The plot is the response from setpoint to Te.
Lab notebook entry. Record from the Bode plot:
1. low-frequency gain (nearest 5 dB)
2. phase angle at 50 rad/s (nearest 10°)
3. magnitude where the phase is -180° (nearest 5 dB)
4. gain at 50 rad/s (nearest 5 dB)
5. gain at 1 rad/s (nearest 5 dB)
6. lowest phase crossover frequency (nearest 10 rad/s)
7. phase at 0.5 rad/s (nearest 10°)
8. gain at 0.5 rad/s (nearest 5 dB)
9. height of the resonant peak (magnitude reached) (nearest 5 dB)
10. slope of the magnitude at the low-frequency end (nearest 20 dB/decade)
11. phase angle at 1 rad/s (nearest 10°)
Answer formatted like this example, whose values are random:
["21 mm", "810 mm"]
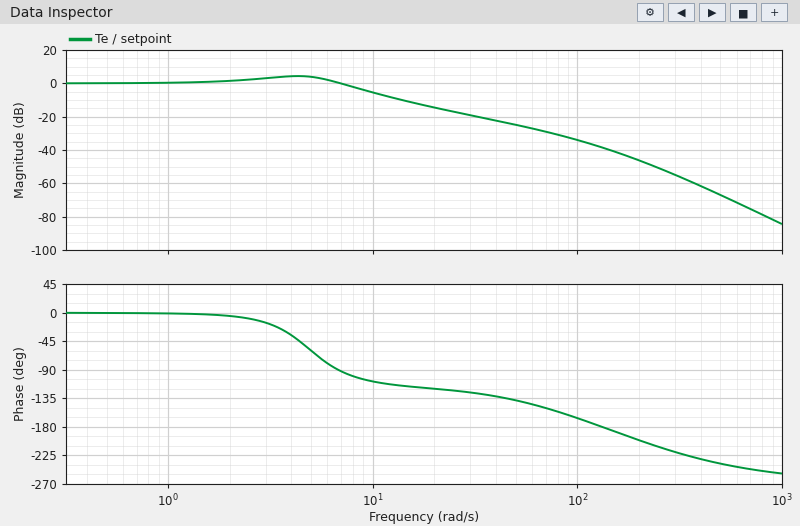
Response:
["0 dB", "-140°", "-40 dB", "-25 dB", "0 dB", "130 rad/s", "0°", "0 dB", "5 dB", "0 dB/decade", "0°"]
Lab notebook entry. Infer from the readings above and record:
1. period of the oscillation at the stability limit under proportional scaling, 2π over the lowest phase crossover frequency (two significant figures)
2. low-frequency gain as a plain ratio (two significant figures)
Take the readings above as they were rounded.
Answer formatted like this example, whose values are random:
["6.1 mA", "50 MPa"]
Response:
["0.048 s", "1.0"]
